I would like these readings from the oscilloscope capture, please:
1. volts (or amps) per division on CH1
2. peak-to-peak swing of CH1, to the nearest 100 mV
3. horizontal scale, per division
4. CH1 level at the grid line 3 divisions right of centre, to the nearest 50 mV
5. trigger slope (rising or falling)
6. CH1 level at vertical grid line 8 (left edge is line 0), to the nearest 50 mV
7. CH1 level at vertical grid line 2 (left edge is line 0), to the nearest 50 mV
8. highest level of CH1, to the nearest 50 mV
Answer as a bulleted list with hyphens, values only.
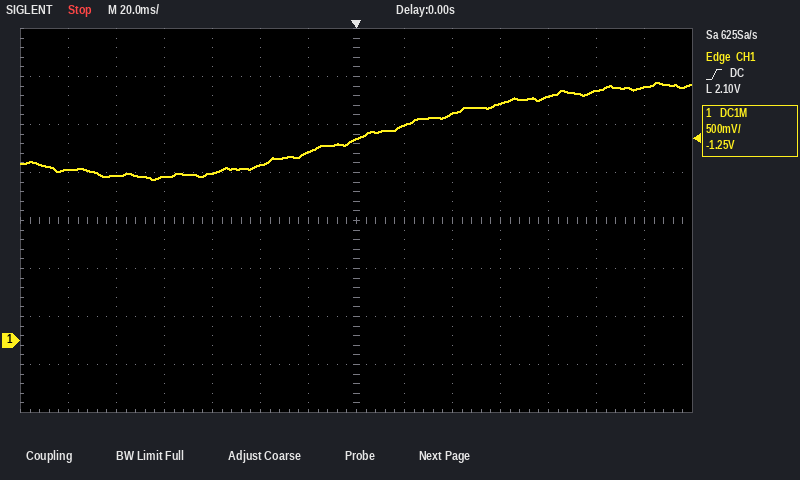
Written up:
- 500 mV
- 1.00 V
- 20 ms
- 2.45 V
- rising
- 2.25 V
- 1.70 V
- 2.70 V
